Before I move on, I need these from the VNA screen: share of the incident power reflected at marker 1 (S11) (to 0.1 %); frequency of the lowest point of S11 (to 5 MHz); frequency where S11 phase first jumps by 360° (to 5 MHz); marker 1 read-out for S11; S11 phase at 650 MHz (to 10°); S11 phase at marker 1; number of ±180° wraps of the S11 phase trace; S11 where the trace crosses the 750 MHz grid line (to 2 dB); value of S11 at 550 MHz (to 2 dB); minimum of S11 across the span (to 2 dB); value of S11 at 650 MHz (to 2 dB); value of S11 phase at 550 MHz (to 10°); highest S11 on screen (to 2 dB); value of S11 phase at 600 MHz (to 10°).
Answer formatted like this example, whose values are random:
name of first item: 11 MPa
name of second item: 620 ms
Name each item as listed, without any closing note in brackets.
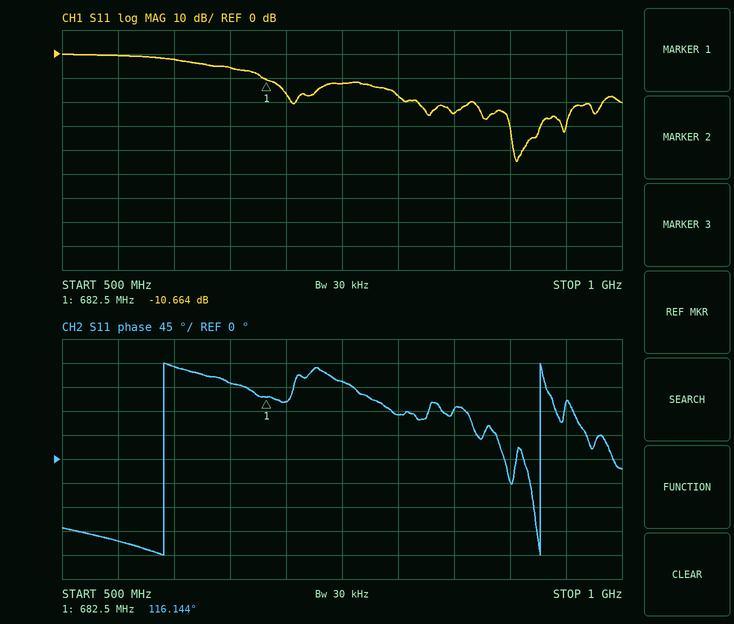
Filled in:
share of the incident power reflected at marker 1 (S11): 8.6 %
frequency of the lowest point of S11: 905 MHz
frequency where S11 phase first jumps by 360°: 590 MHz
marker 1 read-out for S11: -10.664 dB
S11 phase at 650 MHz: 140°
S11 phase at marker 1: 116.144°
number of ±180° wraps of the S11 phase trace: 2
S11 where the trace crosses the 750 MHz grid line: -12 dB
value of S11 at 550 MHz: 0 dB
minimum of S11 across the span: -44 dB
value of S11 at 650 MHz: -6 dB
value of S11 phase at 550 MHz: -150°
highest S11 on screen: 0 dB
value of S11 phase at 600 MHz: 170°
